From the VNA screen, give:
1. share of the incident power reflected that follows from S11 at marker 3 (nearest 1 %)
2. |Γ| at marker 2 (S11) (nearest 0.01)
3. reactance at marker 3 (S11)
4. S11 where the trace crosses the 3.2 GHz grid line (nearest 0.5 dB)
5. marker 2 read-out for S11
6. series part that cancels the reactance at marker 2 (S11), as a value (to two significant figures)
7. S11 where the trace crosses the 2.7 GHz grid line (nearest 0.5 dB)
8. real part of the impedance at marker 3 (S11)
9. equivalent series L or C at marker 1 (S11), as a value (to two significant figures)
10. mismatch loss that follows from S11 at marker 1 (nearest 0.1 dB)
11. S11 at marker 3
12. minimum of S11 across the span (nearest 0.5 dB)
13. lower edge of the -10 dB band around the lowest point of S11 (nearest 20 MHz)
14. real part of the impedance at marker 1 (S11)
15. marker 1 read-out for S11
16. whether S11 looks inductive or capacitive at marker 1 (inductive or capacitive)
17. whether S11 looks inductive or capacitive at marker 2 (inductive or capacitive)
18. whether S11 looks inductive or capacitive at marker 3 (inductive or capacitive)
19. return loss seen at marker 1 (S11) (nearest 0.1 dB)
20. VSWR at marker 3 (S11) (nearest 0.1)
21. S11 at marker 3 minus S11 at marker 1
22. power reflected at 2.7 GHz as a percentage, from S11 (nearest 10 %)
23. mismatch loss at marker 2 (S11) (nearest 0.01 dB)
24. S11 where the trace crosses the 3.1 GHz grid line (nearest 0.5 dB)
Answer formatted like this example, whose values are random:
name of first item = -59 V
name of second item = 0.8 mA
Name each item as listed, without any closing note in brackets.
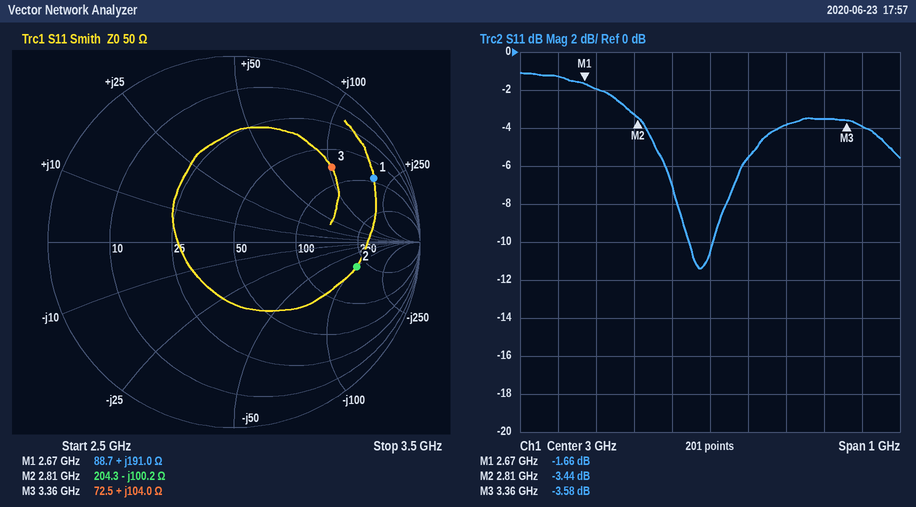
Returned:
share of the incident power reflected that follows from S11 at marker 3 = 44 %
|Γ| at marker 2 (S11) = 0.67
reactance at marker 3 = +104.0 Ω
S11 where the trace crosses the 3.2 GHz grid line = -4.0 dB
marker 2 read-out for S11 = -3.44 dB
series part that cancels the reactance at marker 2 (S11), as a value = 5.7 nH
S11 where the trace crosses the 2.7 GHz grid line = -2.0 dB
real part of the impedance at marker 3 = 72.5 Ω
equivalent series L or C at marker 1 (S11), as a value = 11 nH
mismatch loss that follows from S11 at marker 1 = 5.0 dB
S11 at marker 3 = -3.58 dB
minimum of S11 across the span = -11.5 dB
lower edge of the -10 dB band around the lowest point of S11 = 2.94 GHz
real part of the impedance at marker 1 = 88.7 Ω
marker 1 read-out for S11 = -1.66 dB
whether S11 looks inductive or capacitive at marker 1 = inductive
whether S11 looks inductive or capacitive at marker 2 = capacitive
whether S11 looks inductive or capacitive at marker 3 = inductive
return loss seen at marker 1 (S11) = 1.7 dB
VSWR at marker 3 (S11) = 4.9
S11 at marker 3 minus S11 at marker 1 = -1.92 dB
power reflected at 2.7 GHz as a percentage, from S11 = 60 %
mismatch loss at marker 2 (S11) = 2.62 dB
S11 where the trace crosses the 3.1 GHz grid line = -5.5 dB
